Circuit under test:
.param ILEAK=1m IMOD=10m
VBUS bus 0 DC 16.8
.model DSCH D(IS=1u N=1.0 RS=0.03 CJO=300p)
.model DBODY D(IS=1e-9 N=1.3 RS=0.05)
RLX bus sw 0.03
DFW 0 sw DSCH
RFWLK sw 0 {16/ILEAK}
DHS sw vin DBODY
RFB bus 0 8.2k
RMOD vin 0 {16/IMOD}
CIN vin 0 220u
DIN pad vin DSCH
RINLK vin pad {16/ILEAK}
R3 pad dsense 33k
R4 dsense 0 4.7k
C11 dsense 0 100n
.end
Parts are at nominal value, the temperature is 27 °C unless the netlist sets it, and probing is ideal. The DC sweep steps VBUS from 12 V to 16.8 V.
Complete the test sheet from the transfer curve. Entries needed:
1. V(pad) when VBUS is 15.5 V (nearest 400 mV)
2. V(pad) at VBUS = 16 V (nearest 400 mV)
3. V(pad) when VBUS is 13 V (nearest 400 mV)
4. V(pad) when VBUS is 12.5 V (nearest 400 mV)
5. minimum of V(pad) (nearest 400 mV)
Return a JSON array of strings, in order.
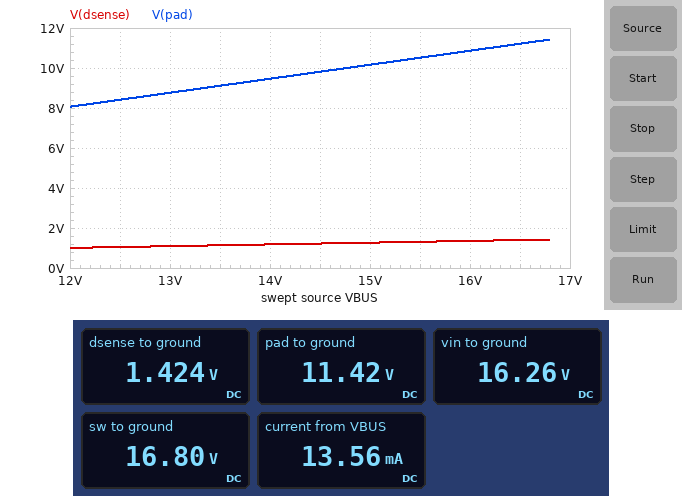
["10.4 V", "10.8 V", "8.8 V", "8.4 V", "8.0 V"]
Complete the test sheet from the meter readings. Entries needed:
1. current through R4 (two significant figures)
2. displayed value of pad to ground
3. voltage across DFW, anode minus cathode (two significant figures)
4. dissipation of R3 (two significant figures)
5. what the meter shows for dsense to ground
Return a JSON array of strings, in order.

["300 µA", "11.42 V", "-17 V", "3.0 mW", "1.424 V"]
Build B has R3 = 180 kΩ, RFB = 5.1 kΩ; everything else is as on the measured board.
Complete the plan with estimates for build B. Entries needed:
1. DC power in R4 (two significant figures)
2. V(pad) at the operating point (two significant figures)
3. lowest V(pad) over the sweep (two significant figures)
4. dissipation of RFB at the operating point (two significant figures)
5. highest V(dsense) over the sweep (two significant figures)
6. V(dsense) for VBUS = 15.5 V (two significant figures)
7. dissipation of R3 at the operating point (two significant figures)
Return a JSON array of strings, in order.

["31 µW", "15 V", "11 V", "55 mW", "380 mV", "350 mV", "1.2 mW"]
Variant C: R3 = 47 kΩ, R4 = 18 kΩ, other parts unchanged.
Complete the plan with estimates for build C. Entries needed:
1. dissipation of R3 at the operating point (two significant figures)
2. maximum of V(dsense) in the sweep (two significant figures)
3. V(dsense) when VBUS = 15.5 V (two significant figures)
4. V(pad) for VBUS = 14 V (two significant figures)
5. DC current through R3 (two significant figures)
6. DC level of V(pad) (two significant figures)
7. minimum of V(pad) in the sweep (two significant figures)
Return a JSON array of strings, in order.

["1.9 mW", "3.6 V", "3.3 V", "11 V", "200 µA", "13 V", "9.2 V"]
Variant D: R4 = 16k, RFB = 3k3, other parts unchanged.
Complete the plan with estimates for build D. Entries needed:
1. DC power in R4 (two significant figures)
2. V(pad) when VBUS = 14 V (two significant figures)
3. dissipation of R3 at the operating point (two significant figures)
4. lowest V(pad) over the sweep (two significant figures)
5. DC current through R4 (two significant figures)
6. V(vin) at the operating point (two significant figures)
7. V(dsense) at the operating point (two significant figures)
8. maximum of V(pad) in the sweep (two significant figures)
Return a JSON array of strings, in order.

["1.0 mW", "10 V", "2.1 mW", "8.7 V", "250 µA", "16 V", "4.0 V", "12 V"]
